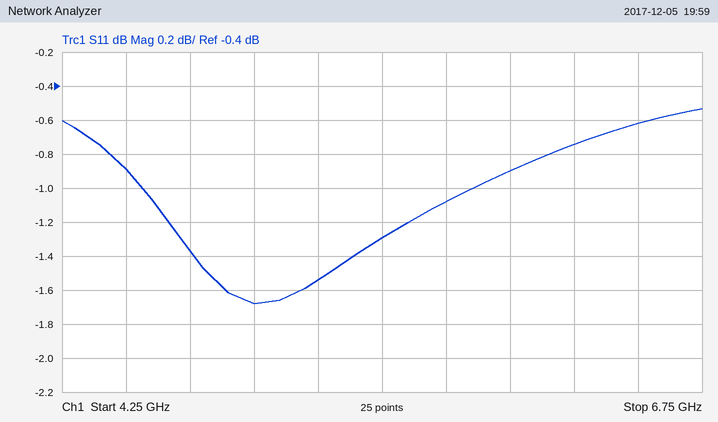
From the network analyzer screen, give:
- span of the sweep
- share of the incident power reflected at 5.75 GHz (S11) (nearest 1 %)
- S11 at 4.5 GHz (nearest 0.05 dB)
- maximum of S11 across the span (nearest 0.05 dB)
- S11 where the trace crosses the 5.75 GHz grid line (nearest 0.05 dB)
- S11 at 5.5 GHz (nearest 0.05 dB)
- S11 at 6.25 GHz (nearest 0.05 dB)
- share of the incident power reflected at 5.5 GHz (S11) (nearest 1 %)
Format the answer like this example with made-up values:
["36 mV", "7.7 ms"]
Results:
["2.5 GHz", "78 %", "-0.90 dB", "-0.55 dB", "-1.10 dB", "-1.30 dB", "-0.75 dB", "74 %"]
